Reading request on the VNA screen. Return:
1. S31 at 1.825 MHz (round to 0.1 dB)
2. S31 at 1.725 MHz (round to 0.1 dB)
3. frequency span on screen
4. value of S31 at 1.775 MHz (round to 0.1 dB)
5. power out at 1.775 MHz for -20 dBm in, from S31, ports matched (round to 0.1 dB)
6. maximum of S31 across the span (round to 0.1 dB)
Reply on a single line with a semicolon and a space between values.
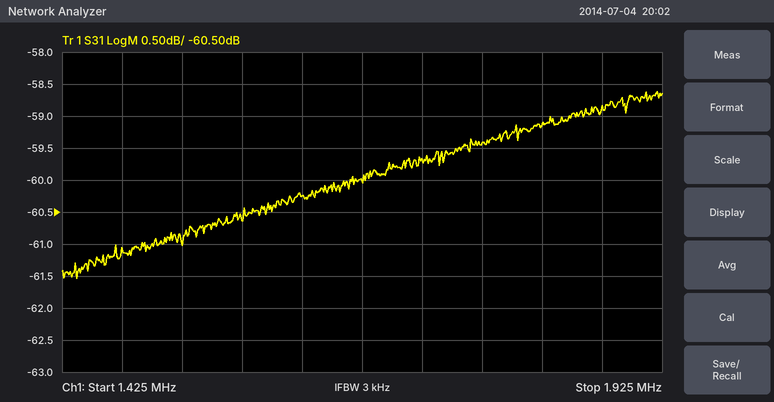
-59.1 dB; -59.7 dB; 500 kHz; -59.4 dB; -79.4 dBm; -58.6 dB
